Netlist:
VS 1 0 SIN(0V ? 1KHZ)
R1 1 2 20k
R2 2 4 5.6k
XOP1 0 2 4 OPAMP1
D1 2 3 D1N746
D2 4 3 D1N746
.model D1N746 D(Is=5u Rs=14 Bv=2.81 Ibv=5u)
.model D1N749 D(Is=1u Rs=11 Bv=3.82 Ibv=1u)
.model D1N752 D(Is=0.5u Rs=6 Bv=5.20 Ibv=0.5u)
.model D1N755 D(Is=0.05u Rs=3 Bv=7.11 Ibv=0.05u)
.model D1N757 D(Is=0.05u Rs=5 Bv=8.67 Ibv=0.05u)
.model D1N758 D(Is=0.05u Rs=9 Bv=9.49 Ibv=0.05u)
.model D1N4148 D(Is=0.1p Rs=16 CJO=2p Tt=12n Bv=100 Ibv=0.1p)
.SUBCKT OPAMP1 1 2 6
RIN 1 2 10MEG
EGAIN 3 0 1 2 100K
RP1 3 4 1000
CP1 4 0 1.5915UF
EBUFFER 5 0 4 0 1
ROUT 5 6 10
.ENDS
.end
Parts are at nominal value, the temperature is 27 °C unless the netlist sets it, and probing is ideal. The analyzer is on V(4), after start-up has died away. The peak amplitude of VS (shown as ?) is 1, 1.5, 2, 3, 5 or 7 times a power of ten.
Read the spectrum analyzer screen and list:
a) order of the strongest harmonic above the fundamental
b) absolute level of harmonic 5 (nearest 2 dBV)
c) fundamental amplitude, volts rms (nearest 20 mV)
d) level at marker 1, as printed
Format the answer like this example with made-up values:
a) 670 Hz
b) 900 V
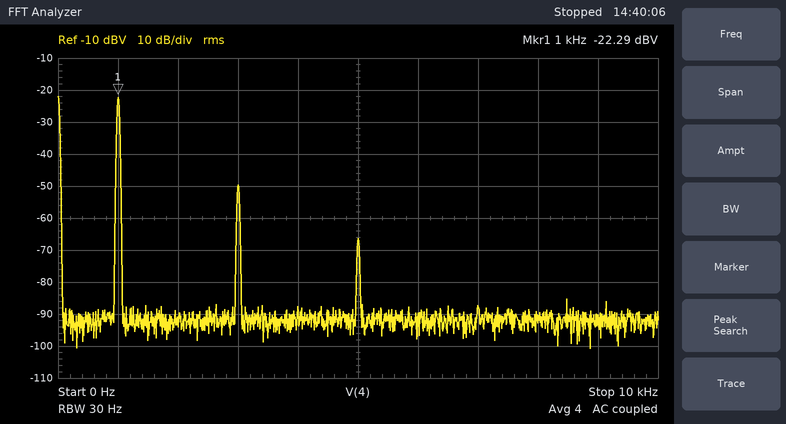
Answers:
a) 3
b) -66 dBV
c) 80 mV
d) -22.29 dBV
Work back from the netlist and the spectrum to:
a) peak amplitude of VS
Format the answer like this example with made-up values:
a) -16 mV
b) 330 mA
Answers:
a) 500 mV
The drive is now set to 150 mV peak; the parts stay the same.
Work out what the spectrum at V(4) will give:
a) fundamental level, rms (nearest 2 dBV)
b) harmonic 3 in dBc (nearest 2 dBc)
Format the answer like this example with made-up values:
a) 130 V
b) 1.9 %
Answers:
a) -34 dBV
b) -42 dBc
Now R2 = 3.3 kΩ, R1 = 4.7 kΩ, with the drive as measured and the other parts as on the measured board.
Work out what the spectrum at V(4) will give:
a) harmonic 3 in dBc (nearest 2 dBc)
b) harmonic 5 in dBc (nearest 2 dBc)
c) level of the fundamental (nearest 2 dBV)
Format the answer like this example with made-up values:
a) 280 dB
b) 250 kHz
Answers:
a) -34 dBc
b) -40 dBc
c) -12 dBV
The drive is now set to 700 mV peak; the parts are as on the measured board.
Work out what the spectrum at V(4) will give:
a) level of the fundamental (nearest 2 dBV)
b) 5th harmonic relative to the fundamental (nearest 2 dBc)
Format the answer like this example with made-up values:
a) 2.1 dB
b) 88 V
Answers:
a) -18 dBV
b) -38 dBc
